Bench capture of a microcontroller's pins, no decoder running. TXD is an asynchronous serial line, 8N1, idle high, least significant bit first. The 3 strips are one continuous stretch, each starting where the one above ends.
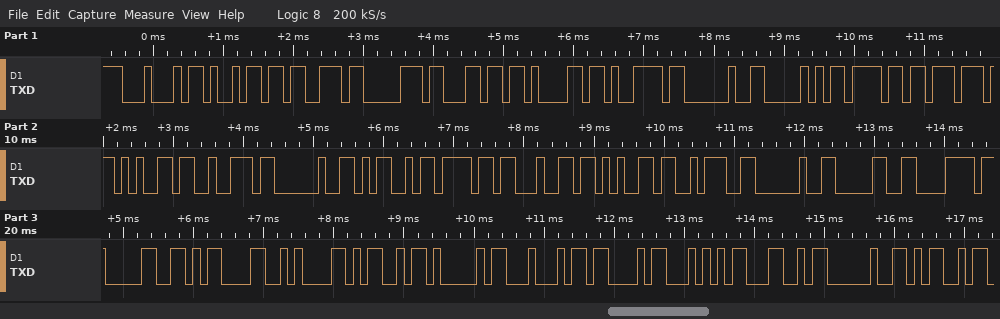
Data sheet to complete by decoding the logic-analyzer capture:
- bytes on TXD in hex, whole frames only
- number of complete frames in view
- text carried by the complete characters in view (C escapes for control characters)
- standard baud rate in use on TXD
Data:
0x44 0x69 0x73 0x70 0x6C 0x61 0x79 0x20 0x50 0x6F 0x77 0x65 0x72 0x20 0x4D 0x6F 0x64 0x65 0x3A 0x20 0x30 0x78 0x30 0x0D 0x0A 0x4D 0x41 0x44 0x43 0x54 0x4C 0x20 0x4D
33
"Display Power Mode: 0x0\r\nMADCTL M"
9600 baud
